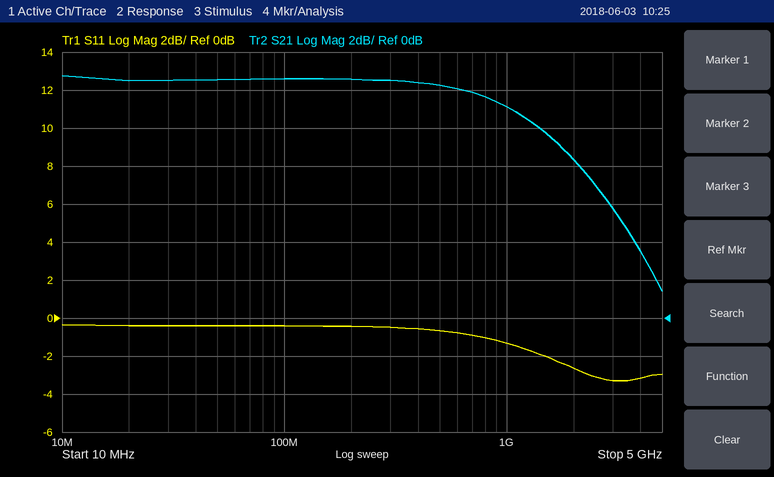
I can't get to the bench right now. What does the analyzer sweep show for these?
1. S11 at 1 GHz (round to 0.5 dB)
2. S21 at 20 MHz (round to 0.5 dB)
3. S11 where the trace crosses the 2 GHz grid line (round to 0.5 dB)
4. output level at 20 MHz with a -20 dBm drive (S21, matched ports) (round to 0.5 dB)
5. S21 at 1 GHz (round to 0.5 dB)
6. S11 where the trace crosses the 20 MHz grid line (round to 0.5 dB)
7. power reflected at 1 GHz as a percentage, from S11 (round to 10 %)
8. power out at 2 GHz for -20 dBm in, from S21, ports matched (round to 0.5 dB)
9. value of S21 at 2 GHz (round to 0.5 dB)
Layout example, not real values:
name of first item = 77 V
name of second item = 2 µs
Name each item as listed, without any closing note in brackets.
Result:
S11 at 1 GHz = -1.5 dB
S21 at 20 MHz = 12.5 dB
S11 where the trace crosses the 2 GHz grid line = -2.5 dB
output level at 20 MHz with a -20 dBm drive (S21, matched ports) = -7.5 dBm
S21 at 1 GHz = 11.0 dB
S11 where the trace crosses the 20 MHz grid line = -0.5 dB
power reflected at 1 GHz as a percentage, from S11 = 70 %
power out at 2 GHz for -20 dBm in, from S21, ports matched = -11.5 dBm
value of S21 at 2 GHz = 8.5 dB
